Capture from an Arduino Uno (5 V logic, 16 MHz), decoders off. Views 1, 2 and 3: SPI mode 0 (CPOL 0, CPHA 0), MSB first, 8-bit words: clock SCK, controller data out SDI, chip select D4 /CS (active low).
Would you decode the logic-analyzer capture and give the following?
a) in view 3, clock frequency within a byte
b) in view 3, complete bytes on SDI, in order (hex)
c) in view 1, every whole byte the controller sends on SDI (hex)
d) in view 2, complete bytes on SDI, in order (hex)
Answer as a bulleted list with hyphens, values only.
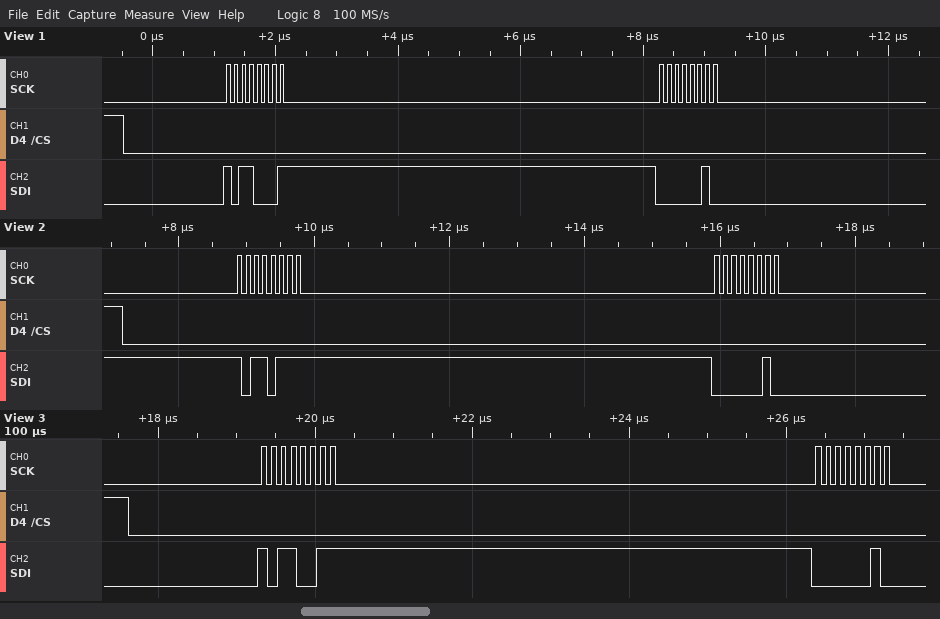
- 8 MHz
- 0xB3 0x02
- B1 02
- 0xB7 0x02
